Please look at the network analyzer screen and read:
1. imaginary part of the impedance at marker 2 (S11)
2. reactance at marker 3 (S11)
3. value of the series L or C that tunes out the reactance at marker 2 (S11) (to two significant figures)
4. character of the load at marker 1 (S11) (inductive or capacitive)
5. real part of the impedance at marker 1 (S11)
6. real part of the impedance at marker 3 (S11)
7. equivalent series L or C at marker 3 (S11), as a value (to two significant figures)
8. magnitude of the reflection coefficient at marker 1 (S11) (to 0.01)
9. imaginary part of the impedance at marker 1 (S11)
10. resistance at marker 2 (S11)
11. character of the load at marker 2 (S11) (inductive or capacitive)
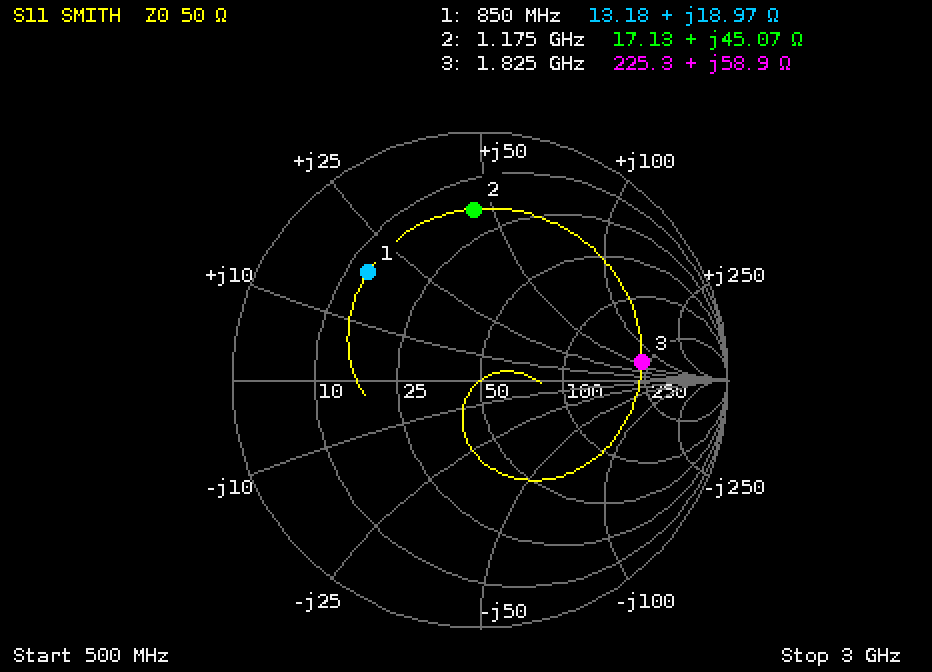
+45.07 Ω
+58.9 Ω
3.0 pF
inductive
13.18 Ω
225.3 Ω
5.1 nH
0.63
+18.97 Ω
17.13 Ω
inductive
